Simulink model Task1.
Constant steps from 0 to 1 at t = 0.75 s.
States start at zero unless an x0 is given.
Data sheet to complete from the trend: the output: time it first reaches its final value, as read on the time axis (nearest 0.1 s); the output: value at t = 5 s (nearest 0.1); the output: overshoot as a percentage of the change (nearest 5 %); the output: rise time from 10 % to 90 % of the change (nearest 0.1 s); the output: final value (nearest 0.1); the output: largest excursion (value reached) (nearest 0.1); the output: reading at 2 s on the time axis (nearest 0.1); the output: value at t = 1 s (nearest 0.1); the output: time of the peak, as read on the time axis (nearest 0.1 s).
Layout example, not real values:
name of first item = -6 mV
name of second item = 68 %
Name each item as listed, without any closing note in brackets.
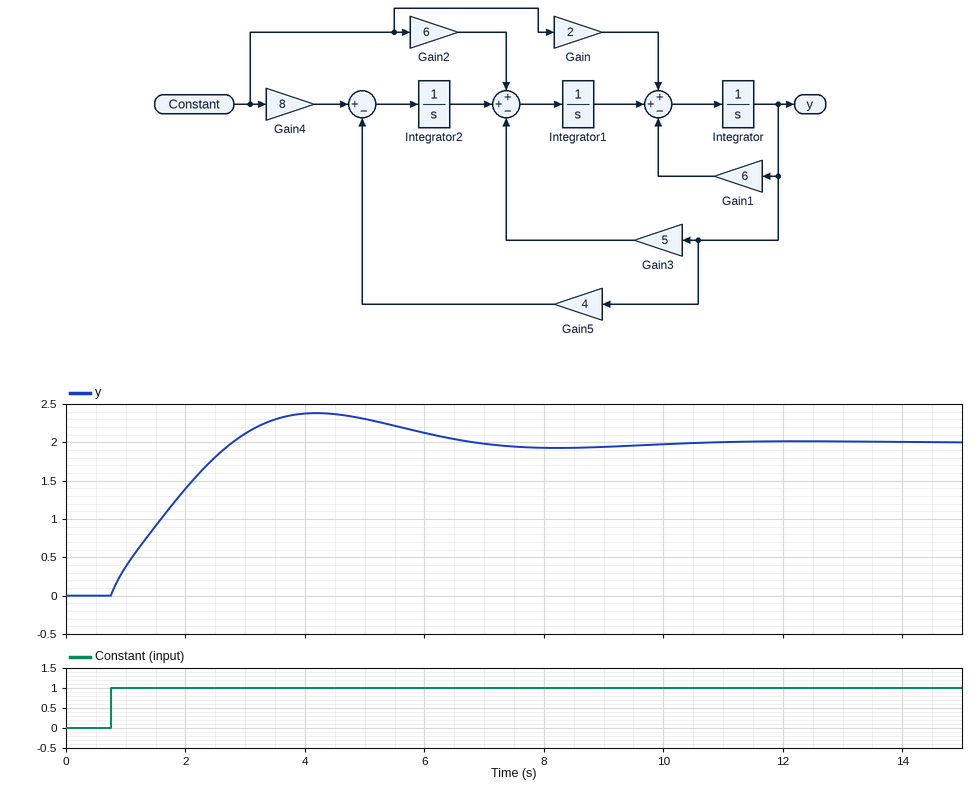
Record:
the output: time it first reaches its final value, as read on the time axis = 2.8 s
the output: value at t = 5 s = 2.3
the output: overshoot as a percentage of the change = 20 %
the output: rise time from 10 % to 90 % of the change = 1.6 s
the output: final value = 2.0
the output: largest excursion (value reached) = 2.4
the output: reading at 2 s on the time axis = 1.4
the output: value at t = 1 s = 0.4
the output: time of the peak, as read on the time axis = 4.2 s
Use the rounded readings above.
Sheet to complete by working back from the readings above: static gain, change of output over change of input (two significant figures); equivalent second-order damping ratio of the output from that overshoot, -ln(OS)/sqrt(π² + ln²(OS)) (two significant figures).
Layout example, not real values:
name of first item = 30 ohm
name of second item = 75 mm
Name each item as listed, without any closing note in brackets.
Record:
static gain, change of output over change of input = 2.0
equivalent second-order damping ratio of the output from that overshoot, -ln(OS)/sqrt(π² + ln²(OS)) = 0.46
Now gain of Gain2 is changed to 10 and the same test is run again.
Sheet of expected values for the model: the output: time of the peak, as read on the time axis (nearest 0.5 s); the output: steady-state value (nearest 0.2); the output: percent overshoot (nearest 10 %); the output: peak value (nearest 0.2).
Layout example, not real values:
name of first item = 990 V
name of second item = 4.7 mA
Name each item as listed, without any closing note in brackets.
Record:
the output: time of the peak, as read on the time axis = 3.5 s
the output: steady-state value = 2.0
the output: percent overshoot = 30 %
the output: peak value = 2.6
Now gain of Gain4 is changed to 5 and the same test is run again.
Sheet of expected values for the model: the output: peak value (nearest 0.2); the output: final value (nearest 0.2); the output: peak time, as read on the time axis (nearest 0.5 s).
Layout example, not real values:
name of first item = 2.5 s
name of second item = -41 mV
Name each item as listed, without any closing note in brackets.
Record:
the output: peak value = 1.6
the output: final value = 1.2
the output: peak time, as read on the time axis = 3.5 s
